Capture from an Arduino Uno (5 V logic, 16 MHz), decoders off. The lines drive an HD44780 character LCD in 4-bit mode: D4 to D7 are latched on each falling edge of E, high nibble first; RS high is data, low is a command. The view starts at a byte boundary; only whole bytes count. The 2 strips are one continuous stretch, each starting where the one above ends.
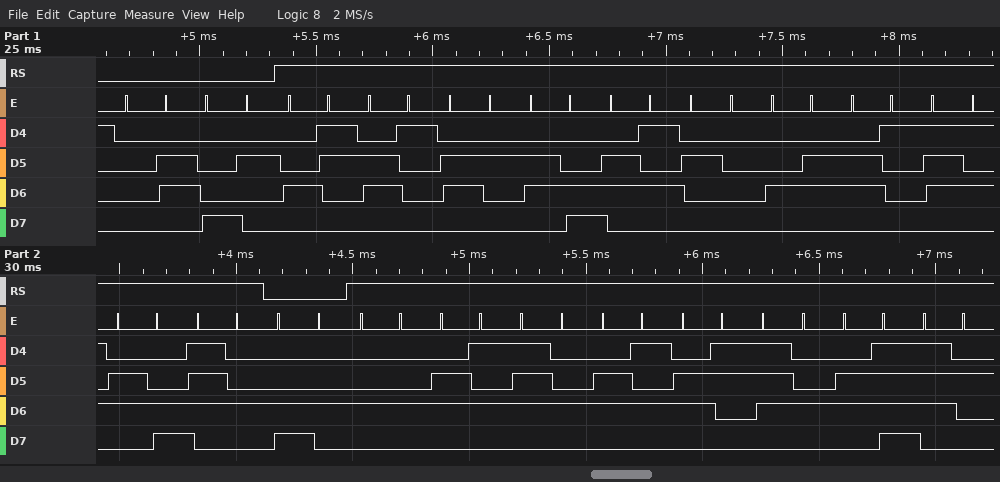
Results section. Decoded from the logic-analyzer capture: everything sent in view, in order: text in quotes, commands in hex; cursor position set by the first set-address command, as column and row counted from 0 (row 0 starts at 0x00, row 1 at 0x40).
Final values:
0x06 0x82 "Cable Fault" 0xC4 "Detector"
column 2, row 0
